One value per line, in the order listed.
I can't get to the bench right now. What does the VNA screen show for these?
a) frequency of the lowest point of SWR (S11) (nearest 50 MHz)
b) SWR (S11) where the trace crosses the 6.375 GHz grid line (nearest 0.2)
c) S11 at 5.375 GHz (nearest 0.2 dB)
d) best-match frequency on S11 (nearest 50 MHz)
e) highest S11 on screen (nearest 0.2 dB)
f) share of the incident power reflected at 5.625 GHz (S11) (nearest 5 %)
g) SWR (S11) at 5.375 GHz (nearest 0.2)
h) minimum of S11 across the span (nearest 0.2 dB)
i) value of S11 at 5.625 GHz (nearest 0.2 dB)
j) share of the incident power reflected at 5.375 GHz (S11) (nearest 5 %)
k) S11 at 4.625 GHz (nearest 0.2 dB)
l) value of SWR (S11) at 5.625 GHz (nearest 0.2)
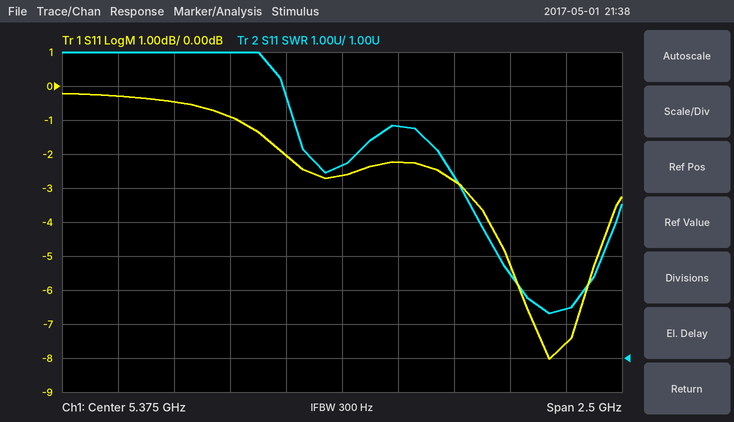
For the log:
6.30 GHz
2.4
-2.6 dB
6.30 GHz
-0.2 dB
60 %
6.6
-8.0 dB
-2.2 dB
55 %
-0.4 dB
7.8
